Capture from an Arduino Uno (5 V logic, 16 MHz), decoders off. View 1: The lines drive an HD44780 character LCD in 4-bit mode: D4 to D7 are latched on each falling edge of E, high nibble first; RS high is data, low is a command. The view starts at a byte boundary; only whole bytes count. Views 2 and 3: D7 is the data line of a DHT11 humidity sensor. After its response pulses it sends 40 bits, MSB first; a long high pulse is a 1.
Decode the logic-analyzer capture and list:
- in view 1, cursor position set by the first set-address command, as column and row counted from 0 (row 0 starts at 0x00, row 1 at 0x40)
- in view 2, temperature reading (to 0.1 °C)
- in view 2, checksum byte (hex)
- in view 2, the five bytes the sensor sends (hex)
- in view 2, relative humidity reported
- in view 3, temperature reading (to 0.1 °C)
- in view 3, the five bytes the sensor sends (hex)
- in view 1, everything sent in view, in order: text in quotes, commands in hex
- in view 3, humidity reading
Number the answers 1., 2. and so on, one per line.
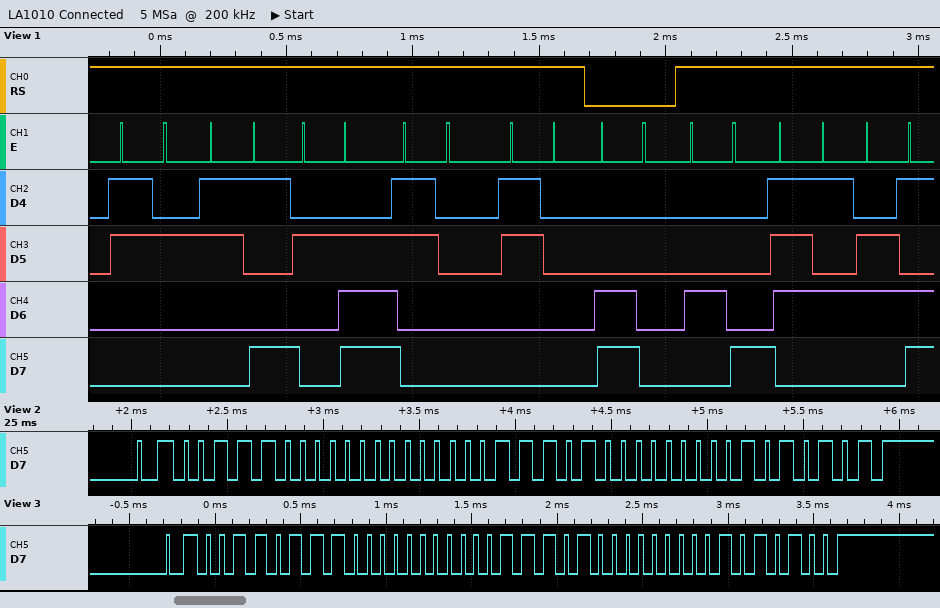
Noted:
1. column 0, row 1
2. 29.0 °C
3. 0x55
4. 38 00 1D 00 55
5. 56 %
6. 29.0 °C
7. 37 00 1D 00 54
8. "29.00" 0xC0 "Hum"
9. 55 %
